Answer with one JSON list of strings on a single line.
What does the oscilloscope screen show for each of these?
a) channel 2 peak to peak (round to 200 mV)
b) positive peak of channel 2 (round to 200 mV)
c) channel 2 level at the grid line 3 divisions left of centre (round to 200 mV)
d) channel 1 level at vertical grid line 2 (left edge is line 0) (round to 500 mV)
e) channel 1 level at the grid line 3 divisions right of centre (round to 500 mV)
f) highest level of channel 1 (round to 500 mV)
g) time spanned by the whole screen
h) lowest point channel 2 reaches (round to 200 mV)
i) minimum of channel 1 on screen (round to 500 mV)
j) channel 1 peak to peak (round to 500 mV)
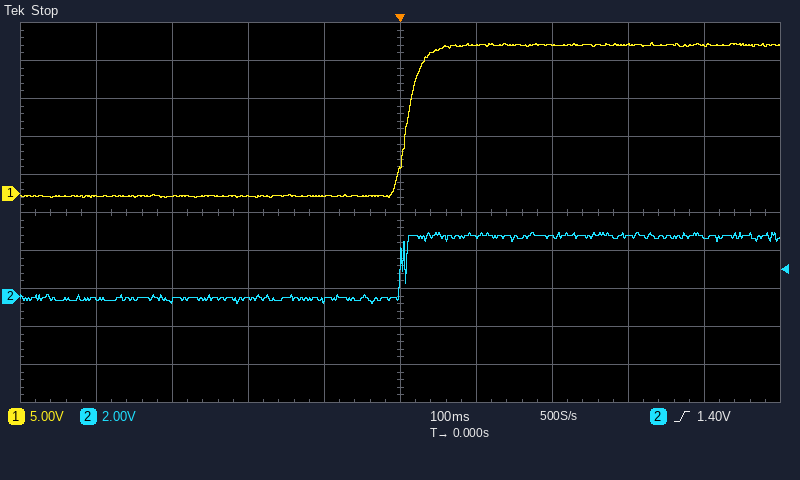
["3.8 V", "3.4 V", "-200 mV", "-500 mV", "19.5 V", "20.0 V", "1 s", "-400 mV", "-500 mV", "20.5 V"]
